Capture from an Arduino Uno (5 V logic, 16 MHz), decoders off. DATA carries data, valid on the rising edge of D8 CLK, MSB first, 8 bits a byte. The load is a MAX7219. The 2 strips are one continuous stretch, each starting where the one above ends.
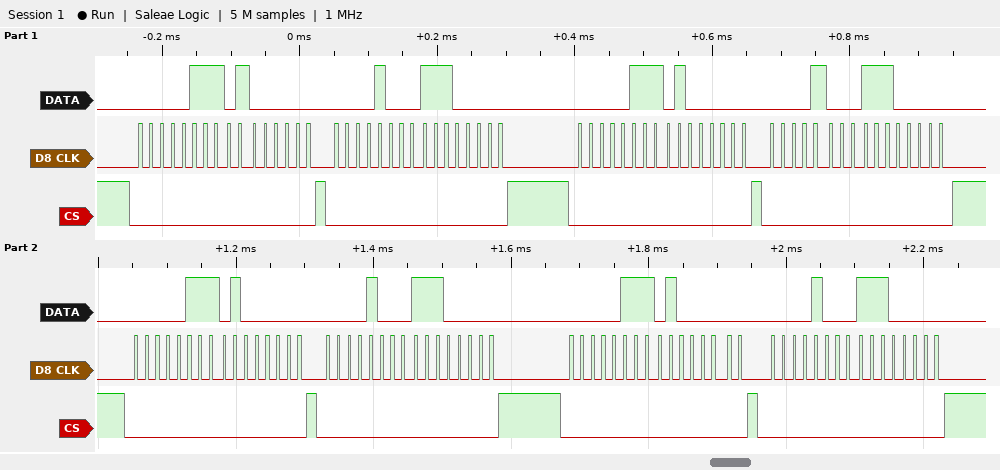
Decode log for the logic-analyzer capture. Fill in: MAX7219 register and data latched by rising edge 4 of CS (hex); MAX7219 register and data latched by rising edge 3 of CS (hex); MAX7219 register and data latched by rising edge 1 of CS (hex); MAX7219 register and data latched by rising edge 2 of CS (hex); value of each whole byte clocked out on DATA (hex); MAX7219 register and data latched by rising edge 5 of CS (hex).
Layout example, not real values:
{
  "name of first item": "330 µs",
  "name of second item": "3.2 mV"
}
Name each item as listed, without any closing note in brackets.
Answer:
{
  "MAX7219 register and data latched by rising edge 4 of CS": "register 0x8, data 0xE0",
  "MAX7219 register and data latched by rising edge 3 of CS": "register 0x7, data 0x40",
  "MAX7219 register and data latched by rising edge 1 of CS": "register 0x7, data 0x40",
  "MAX7219 register and data latched by rising edge 2 of CS": "register 0x8, data 0xE0",
  "value of each whole byte clocked out on DATA": "07 40 08 E0 07 40 08 E0 07 40 08 E0 07 40 08 E0",
  "MAX7219 register and data latched by rising edge 5 of CS": "register 0x7, data 0x40"
}
